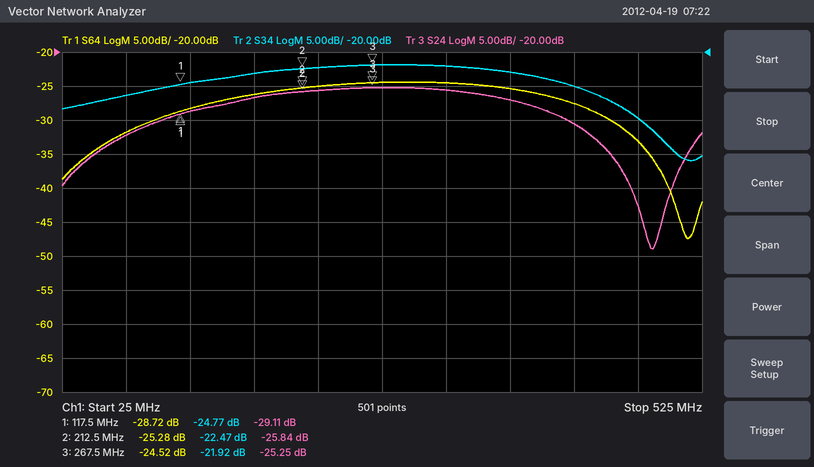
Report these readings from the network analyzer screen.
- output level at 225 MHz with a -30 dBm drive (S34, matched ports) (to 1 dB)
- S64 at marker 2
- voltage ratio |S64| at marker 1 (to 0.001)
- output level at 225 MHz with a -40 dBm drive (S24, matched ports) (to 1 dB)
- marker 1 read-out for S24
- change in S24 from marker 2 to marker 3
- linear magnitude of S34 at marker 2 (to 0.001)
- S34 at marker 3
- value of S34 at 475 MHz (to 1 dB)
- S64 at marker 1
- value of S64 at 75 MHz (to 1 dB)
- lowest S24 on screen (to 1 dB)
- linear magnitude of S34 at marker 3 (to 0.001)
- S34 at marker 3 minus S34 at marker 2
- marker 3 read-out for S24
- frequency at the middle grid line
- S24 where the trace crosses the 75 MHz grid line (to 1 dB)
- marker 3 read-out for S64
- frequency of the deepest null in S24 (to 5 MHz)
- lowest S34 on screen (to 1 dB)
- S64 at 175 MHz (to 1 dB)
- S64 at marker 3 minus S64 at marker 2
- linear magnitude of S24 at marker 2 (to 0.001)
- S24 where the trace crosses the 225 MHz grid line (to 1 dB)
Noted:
-52 dBm
-25.28 dB
0.037
-66 dBm
-29.11 dB
0.59 dB
0.075
-21.92 dB
-30 dB
-28.72 dB
-32 dB
-49 dB
0.080
0.55 dB
-25.25 dB
275 MHz
-32 dB
-24.52 dB
485 MHz
-36 dB
-26 dB
0.76 dB
0.051
-26 dB
